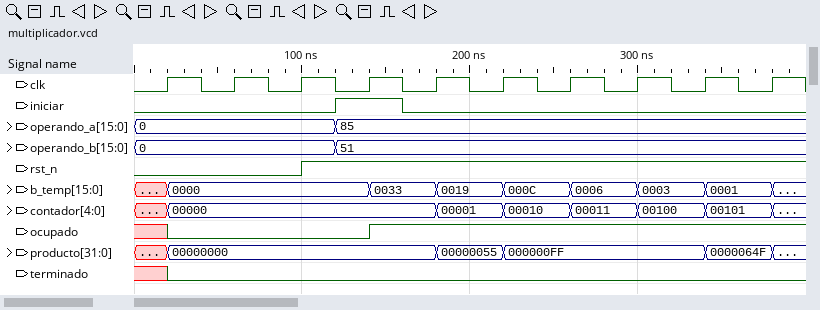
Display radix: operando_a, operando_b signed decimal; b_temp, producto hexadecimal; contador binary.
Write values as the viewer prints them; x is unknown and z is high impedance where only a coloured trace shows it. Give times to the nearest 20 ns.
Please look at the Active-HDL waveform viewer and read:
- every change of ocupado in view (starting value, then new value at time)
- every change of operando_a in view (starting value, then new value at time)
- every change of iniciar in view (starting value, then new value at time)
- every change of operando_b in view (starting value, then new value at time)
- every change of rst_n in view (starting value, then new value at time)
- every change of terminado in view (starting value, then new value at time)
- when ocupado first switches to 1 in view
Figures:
x, 0 at 20 ns, 1 at 140 ns
0, 85 at 120 ns
0, 1 at 120 ns, 0 at 160 ns
0, 51 at 120 ns
0, 1 at 100 ns
x, 0 at 20 ns
140 ns
